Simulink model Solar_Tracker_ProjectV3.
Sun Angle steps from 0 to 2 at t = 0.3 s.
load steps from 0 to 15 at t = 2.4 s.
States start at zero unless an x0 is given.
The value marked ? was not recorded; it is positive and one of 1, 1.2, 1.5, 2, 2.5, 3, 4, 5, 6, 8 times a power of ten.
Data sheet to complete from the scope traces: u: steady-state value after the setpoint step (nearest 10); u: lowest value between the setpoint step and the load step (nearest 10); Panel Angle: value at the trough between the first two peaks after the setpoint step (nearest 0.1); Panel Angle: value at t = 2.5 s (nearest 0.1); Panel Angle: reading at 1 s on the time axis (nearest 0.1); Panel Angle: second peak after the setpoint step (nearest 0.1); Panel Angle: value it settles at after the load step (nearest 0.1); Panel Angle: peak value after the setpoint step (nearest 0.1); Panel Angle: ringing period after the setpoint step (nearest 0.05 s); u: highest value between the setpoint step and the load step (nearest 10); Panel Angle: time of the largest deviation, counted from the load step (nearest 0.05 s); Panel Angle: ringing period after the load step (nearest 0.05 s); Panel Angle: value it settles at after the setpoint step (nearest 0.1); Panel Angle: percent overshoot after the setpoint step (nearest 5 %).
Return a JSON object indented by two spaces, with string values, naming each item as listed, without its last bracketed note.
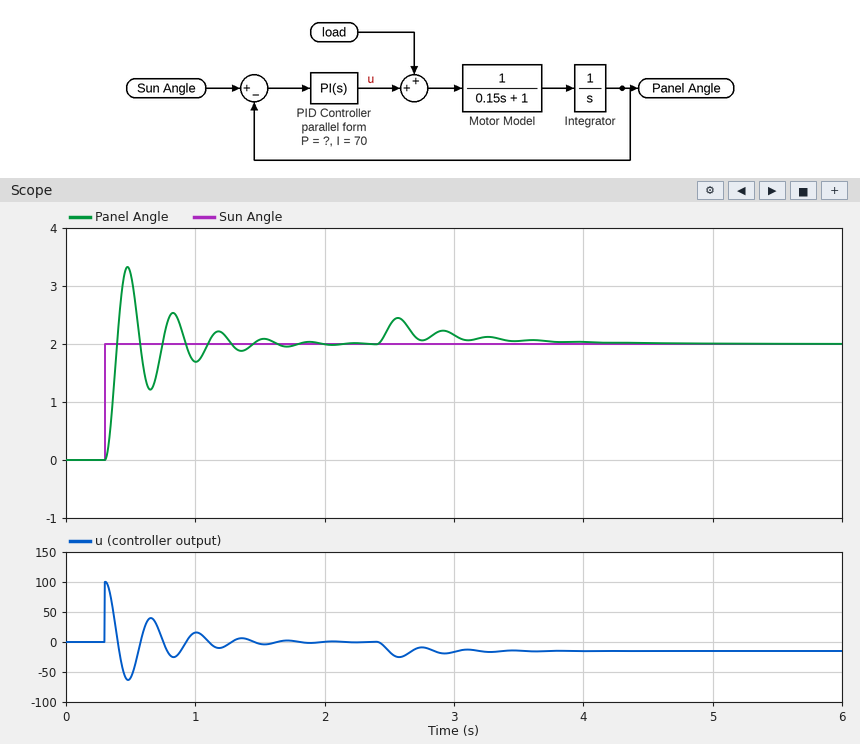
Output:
{
  "u: steady-state value after the setpoint step": "0",
  "u: lowest value between the setpoint step and the load step": "-60",
  "Panel Angle: value at the trough between the first two peaks after the setpoint step": "1.2",
  "Panel Angle: value at t = 2.5 s": "2.3",
  "Panel Angle: reading at 1 s on the time axis": "1.7",
  "Panel Angle: second peak after the setpoint step": "2.5",
  "Panel Angle: value it settles at after the load step": "2.0",
  "Panel Angle: peak value after the setpoint step": "3.3",
  "Panel Angle: ringing period after the setpoint step": "0.35 s",
  "u: highest value between the setpoint step and the load step": "100",
  "Panel Angle: time of the largest deviation, counted from the load step": "0.15 s",
  "Panel Angle: ringing period after the load step": "0.35 s",
  "Panel Angle: value it settles at after the setpoint step": "2.0",
  "Panel Angle: percent overshoot after the setpoint step": "65 %"
}
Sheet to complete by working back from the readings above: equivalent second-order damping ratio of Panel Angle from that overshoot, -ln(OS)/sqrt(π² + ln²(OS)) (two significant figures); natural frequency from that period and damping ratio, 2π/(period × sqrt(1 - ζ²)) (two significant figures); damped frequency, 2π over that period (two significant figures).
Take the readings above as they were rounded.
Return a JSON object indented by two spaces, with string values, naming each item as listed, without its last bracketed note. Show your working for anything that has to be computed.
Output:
{
  "equivalent second-order damping ratio of Panel Angle from that overshoot, -ln(OS)/sqrt(π² + ln²(OS))": "ln(0.65) = -0.431; 0.431 / sqrt(9.870 + 0.186) = 0.14",
  "natural frequency from that period and damping ratio, 2π/(period × sqrt(1 - ζ²))": "2π / (0.35 × sqrt(1 - 0.14²)) = 18 rad/s",
  "damped frequency, 2π over that period": "2π / 0.35 = 18 rad/s"
}
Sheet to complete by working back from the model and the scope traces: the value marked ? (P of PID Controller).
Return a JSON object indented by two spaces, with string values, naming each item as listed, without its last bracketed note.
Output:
{
  "the value marked ?": "50"
}
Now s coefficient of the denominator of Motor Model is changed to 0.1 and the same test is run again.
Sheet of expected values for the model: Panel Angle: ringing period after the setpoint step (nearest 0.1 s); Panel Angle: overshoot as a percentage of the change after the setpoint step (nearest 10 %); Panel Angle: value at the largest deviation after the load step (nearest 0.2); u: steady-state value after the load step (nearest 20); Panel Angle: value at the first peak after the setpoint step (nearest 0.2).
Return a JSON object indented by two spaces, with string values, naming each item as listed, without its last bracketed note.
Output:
{
  "Panel Angle: ringing period after the setpoint step": "0.3 s",
  "Panel Angle: overshoot as a percentage of the change after the setpoint step": "60 %",
  "Panel Angle: value at the largest deviation after the load step": "2.4",
  "u: steady-state value after the load step": "-20",
  "Panel Angle: value at the first peak after the setpoint step": "3.2"
}
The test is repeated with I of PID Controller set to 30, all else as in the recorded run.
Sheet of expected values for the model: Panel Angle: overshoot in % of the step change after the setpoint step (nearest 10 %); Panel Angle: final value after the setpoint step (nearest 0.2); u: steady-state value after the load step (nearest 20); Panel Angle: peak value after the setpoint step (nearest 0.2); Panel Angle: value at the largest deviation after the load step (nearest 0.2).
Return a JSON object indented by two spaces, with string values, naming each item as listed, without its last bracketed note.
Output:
{
  "Panel Angle: overshoot in % of the step change after the setpoint step": "60 %",
  "Panel Angle: final value after the setpoint step": "2.0",
  "u: steady-state value after the load step": "-20",
  "Panel Angle: peak value after the setpoint step": "3.2",
  "Panel Angle: value at the largest deviation after the load step": "2.4"
}
